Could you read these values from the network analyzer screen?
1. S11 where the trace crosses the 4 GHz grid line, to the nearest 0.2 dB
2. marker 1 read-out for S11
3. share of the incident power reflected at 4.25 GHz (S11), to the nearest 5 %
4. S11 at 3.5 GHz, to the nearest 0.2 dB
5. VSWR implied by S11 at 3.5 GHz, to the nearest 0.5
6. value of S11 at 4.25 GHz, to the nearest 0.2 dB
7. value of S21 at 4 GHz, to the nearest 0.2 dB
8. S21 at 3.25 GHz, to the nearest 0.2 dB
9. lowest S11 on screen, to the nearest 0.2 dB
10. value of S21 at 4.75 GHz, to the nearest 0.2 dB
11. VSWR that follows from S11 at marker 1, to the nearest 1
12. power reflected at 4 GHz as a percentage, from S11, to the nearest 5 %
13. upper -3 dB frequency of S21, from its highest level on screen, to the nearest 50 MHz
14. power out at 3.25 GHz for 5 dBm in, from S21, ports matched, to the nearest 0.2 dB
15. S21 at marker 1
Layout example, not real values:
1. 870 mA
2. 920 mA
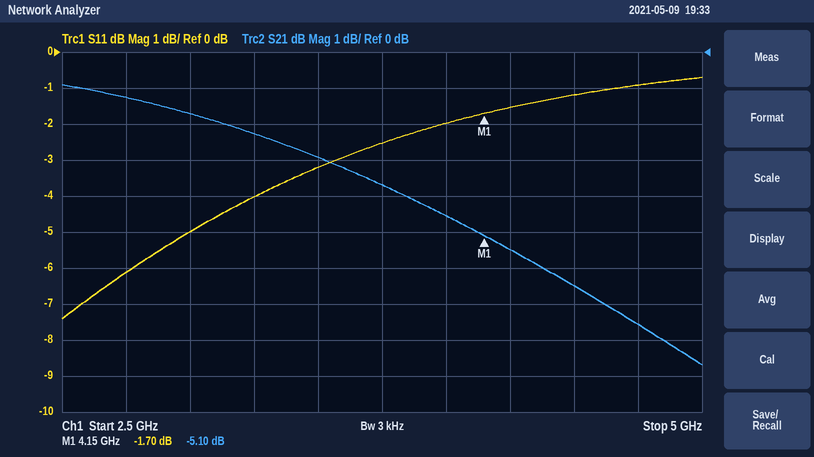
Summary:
1. -2.0 dB
2. -1.70 dB
3. 70 %
4. -3.2 dB
5. 5.5
6. -1.6 dB
7. -4.6 dB
8. -2.2 dB
9. -7.4 dB
10. -7.6 dB
11. 10
12. 65 %
13. 3.80 GHz
14. 2.8 dBm
15. -5.10 dB
